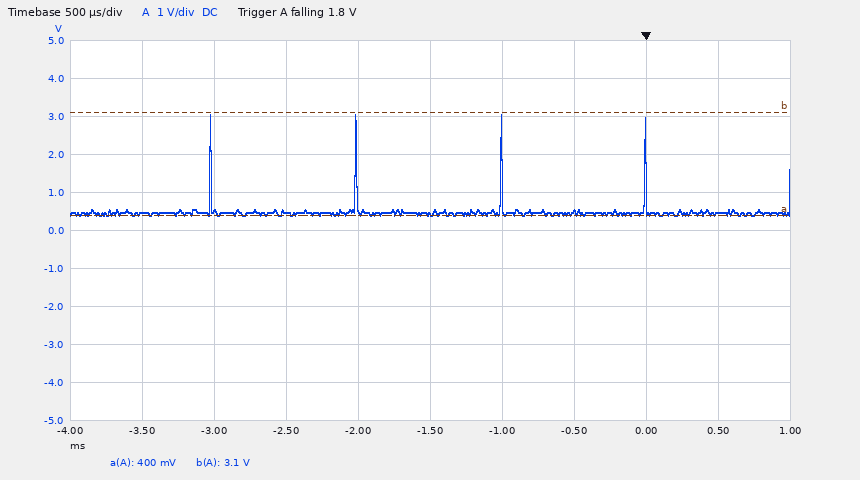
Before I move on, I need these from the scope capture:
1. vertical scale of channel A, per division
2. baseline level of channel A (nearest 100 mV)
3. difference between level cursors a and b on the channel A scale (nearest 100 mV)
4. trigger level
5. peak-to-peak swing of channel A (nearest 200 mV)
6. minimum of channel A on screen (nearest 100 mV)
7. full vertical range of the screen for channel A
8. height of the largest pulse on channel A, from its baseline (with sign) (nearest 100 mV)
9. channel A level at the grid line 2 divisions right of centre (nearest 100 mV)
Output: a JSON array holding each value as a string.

["1 V", "500 mV", "2.7 V", "1.8 V", "2.6 V", "400 mV", "10 V", "+2.6 V", "500 mV"]
